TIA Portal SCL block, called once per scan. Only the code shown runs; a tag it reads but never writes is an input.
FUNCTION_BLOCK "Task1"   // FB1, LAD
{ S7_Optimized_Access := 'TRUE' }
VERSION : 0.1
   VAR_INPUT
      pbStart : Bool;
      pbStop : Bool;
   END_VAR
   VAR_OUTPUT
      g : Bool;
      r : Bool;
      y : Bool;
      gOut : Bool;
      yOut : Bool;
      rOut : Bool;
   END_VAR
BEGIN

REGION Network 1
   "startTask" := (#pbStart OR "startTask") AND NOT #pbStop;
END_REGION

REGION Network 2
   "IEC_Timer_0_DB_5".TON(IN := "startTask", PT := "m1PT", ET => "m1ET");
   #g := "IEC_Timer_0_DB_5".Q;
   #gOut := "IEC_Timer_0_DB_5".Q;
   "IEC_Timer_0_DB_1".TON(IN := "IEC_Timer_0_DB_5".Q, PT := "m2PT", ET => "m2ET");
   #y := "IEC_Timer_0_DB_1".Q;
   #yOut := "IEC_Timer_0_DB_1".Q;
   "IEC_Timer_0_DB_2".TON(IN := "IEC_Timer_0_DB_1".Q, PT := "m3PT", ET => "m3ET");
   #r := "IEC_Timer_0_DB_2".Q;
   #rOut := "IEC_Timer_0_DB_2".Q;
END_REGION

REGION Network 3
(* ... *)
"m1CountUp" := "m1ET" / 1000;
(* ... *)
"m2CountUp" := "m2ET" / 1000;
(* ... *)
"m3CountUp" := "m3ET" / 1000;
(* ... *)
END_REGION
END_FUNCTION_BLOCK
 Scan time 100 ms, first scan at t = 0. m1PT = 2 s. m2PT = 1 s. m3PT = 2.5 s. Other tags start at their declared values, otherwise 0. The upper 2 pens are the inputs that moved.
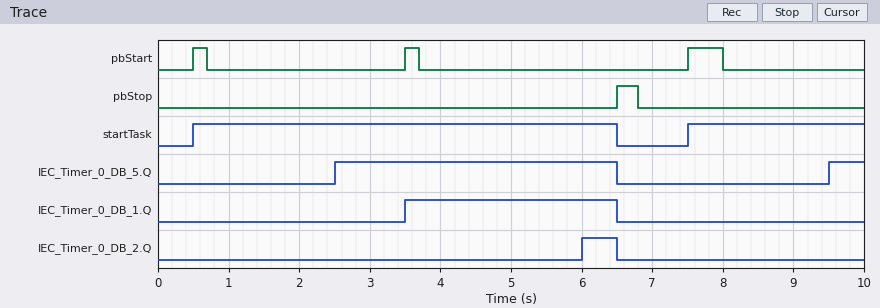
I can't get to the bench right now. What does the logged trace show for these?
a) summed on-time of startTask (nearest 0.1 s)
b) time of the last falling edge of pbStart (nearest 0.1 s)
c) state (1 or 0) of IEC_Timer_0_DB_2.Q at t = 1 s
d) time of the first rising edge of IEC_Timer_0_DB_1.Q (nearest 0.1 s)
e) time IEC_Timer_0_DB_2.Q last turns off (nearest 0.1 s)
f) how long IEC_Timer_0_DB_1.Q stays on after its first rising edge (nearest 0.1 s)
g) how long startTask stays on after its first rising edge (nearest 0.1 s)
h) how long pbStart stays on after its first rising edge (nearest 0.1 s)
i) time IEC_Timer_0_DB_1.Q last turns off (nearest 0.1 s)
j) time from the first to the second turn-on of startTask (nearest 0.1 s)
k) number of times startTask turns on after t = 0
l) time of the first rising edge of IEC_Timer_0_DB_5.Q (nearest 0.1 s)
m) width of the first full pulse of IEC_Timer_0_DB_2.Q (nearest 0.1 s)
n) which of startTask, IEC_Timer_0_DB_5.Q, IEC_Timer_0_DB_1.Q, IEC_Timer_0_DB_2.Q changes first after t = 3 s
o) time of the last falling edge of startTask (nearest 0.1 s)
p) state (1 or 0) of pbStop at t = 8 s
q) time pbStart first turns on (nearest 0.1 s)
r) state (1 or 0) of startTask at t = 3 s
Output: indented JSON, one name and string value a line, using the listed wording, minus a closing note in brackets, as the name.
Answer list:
{
  "summed on-time of startTask": "8.5 s",
  "time of the last falling edge of pbStart": "8.0 s",
  "state (1 or 0) of IEC_Timer_0_DB_2.Q at t = 1 s": "0",
  "time of the first rising edge of IEC_Timer_0_DB_1.Q": "3.5 s",
  "time IEC_Timer_0_DB_2.Q last turns off": "6.5 s",
  "how long IEC_Timer_0_DB_1.Q stays on after its first rising edge": "3.0 s",
  "how long startTask stays on after its first rising edge": "6.0 s",
  "how long pbStart stays on after its first rising edge": "0.2 s",
  "time IEC_Timer_0_DB_1.Q last turns off": "6.5 s",
  "time from the first to the second turn-on of startTask": "7.0 s",
  "number of times startTask turns on after t = 0": "2",
  "time of the first rising edge of IEC_Timer_0_DB_5.Q": "2.5 s",
  "width of the first full pulse of IEC_Timer_0_DB_2.Q": "0.5 s",
  "which of startTask, IEC_Timer_0_DB_5.Q, IEC_Timer_0_DB_1.Q, IEC_Timer_0_DB_2.Q changes first after t = 3 s": "IEC_Timer_0_DB_1.Q",
  "time of the last falling edge of startTask": "6.5 s",
  "state (1 or 0) of pbStop at t = 8 s": "0",
  "time pbStart first turns on": "0.5 s",
  "state (1 or 0) of startTask at t = 3 s": "1"
}
